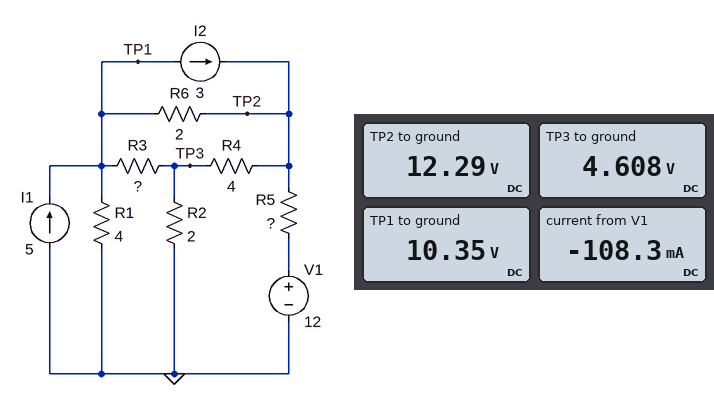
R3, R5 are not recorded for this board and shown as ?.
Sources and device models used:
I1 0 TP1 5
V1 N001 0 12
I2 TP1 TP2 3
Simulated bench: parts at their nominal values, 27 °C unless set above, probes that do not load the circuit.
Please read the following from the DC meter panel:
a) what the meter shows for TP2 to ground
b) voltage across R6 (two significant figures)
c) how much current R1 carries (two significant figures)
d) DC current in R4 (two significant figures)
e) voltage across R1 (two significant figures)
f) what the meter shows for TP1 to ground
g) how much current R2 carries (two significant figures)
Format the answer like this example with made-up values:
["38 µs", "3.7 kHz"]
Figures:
["12.29 V", "1.9 V", "2.6 A", "1.9 A", "10 V", "10.35 V", "2.3 A"]
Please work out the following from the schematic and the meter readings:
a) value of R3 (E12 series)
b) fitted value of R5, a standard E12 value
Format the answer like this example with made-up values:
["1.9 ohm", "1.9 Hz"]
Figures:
["15 Ω", "2.7 Ω"]
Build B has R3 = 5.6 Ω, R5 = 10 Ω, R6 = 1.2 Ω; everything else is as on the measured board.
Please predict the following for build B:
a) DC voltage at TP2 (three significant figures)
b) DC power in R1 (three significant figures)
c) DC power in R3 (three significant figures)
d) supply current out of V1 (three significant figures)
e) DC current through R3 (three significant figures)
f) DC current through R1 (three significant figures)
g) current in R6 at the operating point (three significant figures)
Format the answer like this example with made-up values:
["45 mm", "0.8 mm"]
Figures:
["11.7 V", "25.0 W", "4.36 W", "33.5 mA", "882 mA", "2.50 A", "1.38 A"]
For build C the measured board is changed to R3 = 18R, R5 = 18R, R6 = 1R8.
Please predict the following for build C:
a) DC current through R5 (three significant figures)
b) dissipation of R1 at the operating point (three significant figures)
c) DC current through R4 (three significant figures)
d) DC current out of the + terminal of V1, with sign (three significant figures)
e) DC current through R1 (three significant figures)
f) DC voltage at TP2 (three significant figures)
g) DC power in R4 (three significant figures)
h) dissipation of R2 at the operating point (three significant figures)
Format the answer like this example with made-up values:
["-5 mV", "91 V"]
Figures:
["26.8 mA", "28.5 W", "1.97 A", "-26.8 mA", "2.67 A", "12.5 V", "15.5 W", "10.6 W"]
